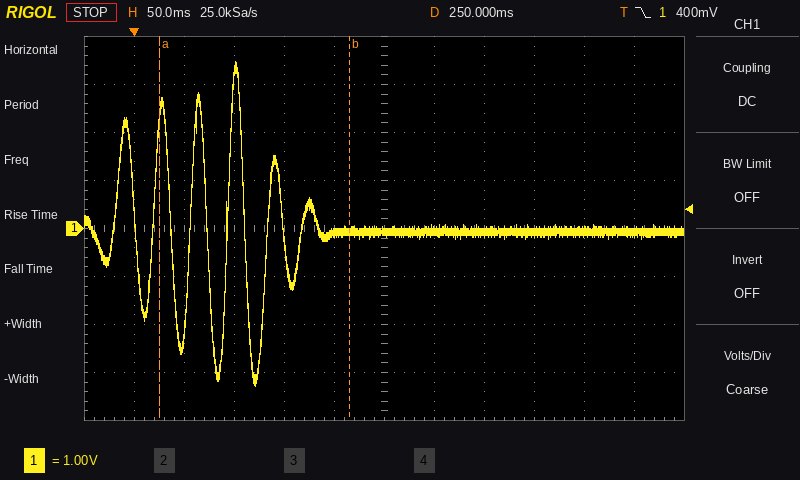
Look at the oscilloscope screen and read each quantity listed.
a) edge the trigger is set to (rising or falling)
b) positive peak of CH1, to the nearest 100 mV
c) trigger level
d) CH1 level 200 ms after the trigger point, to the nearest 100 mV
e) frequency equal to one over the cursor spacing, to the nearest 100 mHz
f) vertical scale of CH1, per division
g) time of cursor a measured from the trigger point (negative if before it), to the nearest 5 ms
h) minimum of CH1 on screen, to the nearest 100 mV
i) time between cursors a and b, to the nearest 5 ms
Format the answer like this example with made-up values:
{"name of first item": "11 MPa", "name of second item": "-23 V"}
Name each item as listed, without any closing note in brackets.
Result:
{"edge the trigger is set to": "falling", "positive peak of CH1, to the nearest 100 mV": "3.5 V", "trigger level": "400 mV", "CH1 level 200 ms after the trigger point, to the nearest 100 mV": "-100 mV", "frequency equal to one over the cursor spacing, to the nearest 100 mHz": "5.3 Hz", "vertical scale of CH1, per division": "1 V", "time of cursor a measured from the trigger point (negative if before it), to the nearest 5 ms": "+25 ms", "minimum of CH1 on screen, to the nearest 100 mV": "-3.3 V", "time between cursors a and b, to the nearest 5 ms": "190 ms"}
